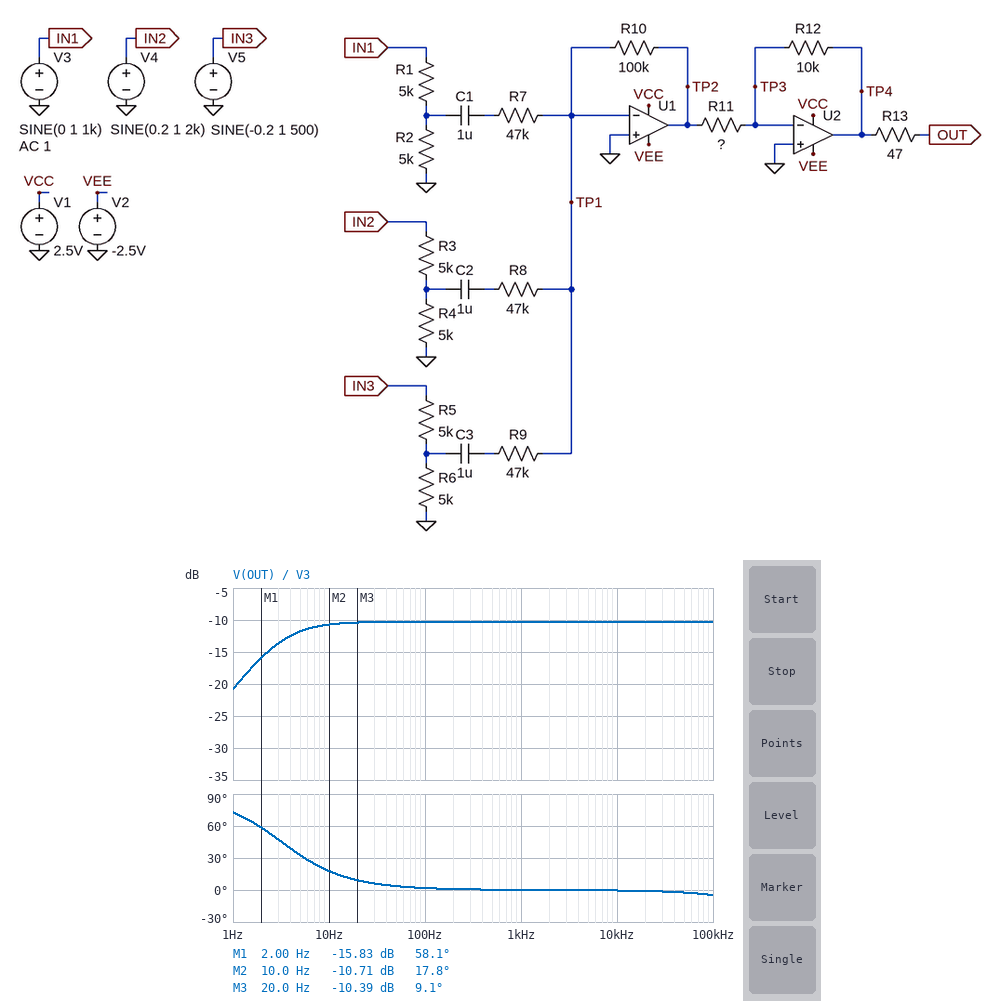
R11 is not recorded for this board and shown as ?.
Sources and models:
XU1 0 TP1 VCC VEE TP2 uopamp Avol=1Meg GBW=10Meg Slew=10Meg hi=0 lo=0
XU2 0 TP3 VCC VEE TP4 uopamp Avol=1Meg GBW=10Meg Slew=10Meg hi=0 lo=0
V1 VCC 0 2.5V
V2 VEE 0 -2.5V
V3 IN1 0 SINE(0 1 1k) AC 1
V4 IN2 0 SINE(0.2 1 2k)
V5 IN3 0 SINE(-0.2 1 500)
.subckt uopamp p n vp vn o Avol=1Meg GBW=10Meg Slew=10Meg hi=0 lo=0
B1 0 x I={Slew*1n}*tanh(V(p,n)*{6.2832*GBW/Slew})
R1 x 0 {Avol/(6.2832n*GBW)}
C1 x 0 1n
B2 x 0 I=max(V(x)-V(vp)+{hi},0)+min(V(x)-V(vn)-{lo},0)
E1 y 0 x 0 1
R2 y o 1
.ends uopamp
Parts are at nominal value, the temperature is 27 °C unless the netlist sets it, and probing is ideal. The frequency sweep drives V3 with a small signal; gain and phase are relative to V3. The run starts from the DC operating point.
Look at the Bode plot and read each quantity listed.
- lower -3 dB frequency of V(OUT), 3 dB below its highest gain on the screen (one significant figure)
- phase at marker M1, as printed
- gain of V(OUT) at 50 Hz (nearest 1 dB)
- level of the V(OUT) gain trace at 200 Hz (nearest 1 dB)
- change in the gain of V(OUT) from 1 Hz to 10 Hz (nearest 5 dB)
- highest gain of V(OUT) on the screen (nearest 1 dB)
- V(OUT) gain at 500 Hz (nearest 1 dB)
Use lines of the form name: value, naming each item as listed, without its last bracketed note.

lower -3 dB frequency of V(OUT), 3 dB below its highest gain on the screen: 3 Hz
phase at marker M1, as printed: 58.1 deg
gain of V(OUT) at 50 Hz: -10 dB
level of the V(OUT) gain trace at 200 Hz: -10 dB
change in the gain of V(OUT) from 1 Hz to 10 Hz: 10 dB
highest gain of V(OUT) on the screen: -10 dB
V(OUT) gain at 500 Hz: -10 dB
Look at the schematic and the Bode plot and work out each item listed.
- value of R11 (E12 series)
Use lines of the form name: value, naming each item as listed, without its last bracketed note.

value of R11: 33 kΩ
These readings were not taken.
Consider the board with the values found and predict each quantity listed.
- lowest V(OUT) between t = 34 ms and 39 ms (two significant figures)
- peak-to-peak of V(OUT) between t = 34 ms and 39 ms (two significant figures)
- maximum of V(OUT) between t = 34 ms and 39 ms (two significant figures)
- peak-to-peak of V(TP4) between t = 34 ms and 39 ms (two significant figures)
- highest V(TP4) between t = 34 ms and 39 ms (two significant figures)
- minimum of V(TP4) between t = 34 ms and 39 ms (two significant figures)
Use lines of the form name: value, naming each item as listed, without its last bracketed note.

lowest V(OUT) between t = 34 ms and 39 ms: -680 mV
peak-to-peak of V(OUT) between t = 34 ms and 39 ms: 1.4 V
maximum of V(OUT) between t = 34 ms and 39 ms: 680 mV
peak-to-peak of V(TP4) between t = 34 ms and 39 ms: 1.4 V
highest V(TP4) between t = 34 ms and 39 ms: 680 mV
minimum of V(TP4) between t = 34 ms and 39 ms: -680 mV
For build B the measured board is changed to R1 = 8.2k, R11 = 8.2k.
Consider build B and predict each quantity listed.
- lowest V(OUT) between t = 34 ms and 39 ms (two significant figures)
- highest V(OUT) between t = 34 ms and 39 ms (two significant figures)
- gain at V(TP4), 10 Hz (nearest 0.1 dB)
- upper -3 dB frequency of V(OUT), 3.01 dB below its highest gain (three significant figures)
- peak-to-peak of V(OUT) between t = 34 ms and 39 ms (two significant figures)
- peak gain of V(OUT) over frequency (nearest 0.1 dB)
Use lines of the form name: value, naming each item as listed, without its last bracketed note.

lowest V(OUT) between t = 34 ms and 39 ms: -2.5 V
highest V(OUT) between t = 34 ms and 39 ms: 2.5 V
gain at V(TP4), 10 Hz: -1.1 dB
upper -3 dB frequency of V(OUT), 3.01 dB below its highest gain: 1.31 MHz
peak-to-peak of V(OUT) between t = 34 ms and 39 ms: 5.0 V
peak gain of V(OUT) over frequency: -0.7 dB
